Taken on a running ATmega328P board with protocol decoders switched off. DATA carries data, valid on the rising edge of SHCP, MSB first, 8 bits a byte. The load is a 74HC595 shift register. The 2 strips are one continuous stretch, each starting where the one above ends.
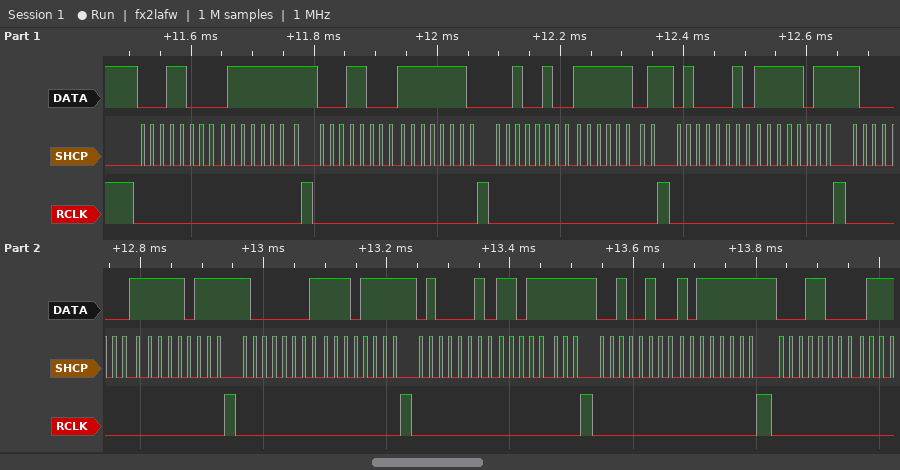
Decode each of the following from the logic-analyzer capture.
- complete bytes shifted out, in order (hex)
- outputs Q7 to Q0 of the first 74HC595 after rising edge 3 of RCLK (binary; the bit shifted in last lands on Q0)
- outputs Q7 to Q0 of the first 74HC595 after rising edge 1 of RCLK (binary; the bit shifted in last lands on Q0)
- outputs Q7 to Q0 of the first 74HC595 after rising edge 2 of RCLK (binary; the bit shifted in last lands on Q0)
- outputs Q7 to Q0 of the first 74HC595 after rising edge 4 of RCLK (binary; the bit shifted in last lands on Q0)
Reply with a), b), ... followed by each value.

a) 18 7F 18 FE 24 FD 42 FB 81 F7 81 EF 42 DF 24 BF 18
b) 11111101
c) 01111111
d) 11111110
e) 11111011
